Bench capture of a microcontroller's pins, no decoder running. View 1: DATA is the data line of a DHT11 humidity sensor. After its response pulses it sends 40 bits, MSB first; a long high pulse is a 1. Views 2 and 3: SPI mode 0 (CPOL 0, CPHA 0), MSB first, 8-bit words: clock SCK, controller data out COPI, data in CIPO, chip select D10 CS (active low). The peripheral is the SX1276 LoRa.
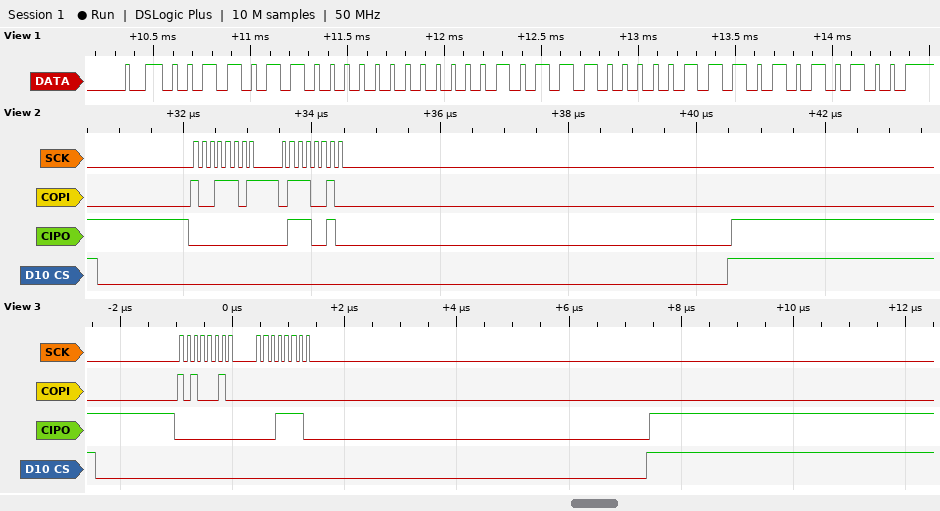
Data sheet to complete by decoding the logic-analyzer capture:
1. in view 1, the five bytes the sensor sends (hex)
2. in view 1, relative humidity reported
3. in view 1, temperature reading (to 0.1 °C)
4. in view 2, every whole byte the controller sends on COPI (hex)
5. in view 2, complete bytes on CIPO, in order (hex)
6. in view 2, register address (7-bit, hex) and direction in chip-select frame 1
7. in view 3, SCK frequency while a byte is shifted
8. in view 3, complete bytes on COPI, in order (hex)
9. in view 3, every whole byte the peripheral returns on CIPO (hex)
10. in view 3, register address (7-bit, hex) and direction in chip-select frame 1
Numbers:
36 00 17 07 54
54 %
23.7 °C
0x9D 0x72
0x00 0x72
0x1D write
8 MHz
A2 00
00 1E
0x22 write
